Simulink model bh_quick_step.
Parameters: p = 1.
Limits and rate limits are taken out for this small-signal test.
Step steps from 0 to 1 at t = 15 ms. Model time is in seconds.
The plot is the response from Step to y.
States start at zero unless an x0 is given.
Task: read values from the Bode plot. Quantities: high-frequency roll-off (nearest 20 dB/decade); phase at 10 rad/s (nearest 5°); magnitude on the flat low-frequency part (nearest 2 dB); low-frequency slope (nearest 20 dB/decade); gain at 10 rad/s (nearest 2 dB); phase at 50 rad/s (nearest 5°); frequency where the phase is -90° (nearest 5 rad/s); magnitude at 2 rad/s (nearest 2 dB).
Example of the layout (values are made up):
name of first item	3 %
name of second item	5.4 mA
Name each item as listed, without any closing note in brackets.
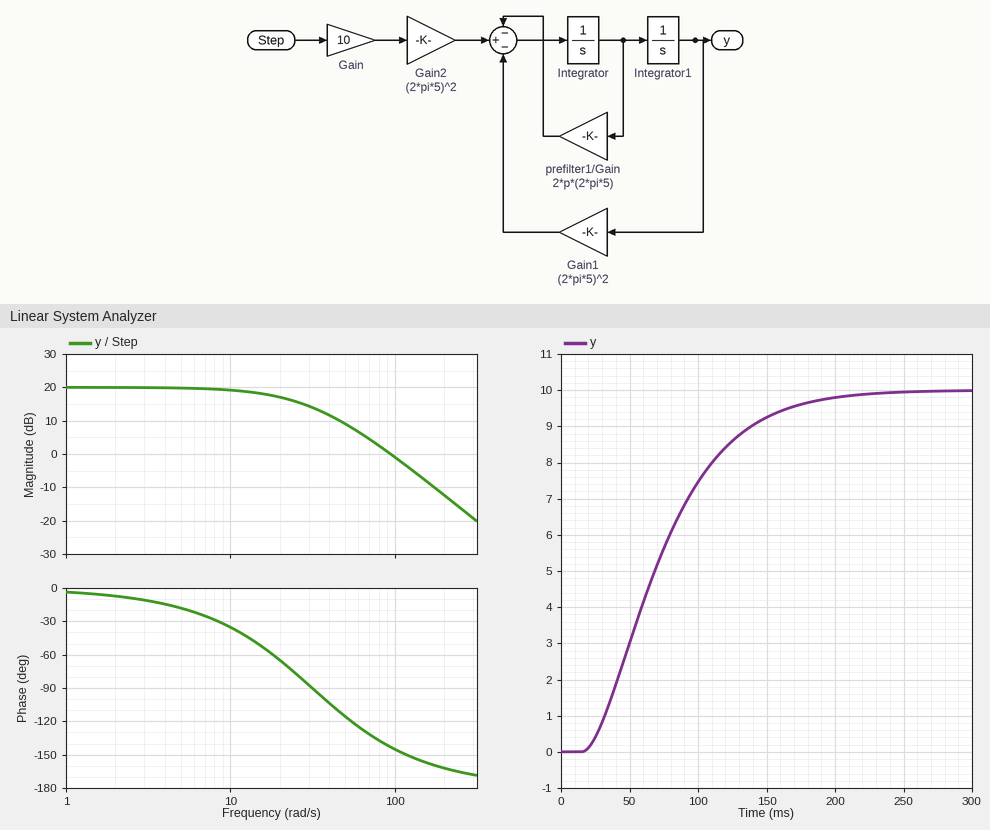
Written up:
high-frequency roll-off	-40 dB/decade
phase at 10 rad/s	-35°
magnitude on the flat low-frequency part	20 dB
low-frequency slope	0 dB/decade
gain at 10 rad/s	20 dB
phase at 50 rad/s	-115°
frequency where the phase is -90°	30 rad/s
magnitude at 2 rad/s	20 dB
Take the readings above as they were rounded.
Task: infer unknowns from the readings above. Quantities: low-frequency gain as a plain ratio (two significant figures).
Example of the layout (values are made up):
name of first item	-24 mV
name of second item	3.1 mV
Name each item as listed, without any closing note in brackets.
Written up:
low-frequency gain as a plain ratio	10
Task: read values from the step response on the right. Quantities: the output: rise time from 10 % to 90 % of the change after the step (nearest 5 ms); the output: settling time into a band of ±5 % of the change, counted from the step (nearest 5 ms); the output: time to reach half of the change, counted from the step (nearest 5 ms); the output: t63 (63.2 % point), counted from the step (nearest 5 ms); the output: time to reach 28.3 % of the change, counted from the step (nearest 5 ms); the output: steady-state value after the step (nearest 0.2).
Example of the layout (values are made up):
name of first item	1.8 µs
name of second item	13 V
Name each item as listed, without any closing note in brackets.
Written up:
the output: rise time from 10 % to 90 % of the change after the step	105 ms
the output: settling time into a band of ±5 % of the change, counted from the step	150 ms
the output: time to reach half of the change, counted from the step	55 ms
the output: t63 (63.2 % point), counted from the step	70 ms
the output: time to reach 28.3 % of the change, counted from the step	35 ms
the output: steady-state value after the step	10.0
